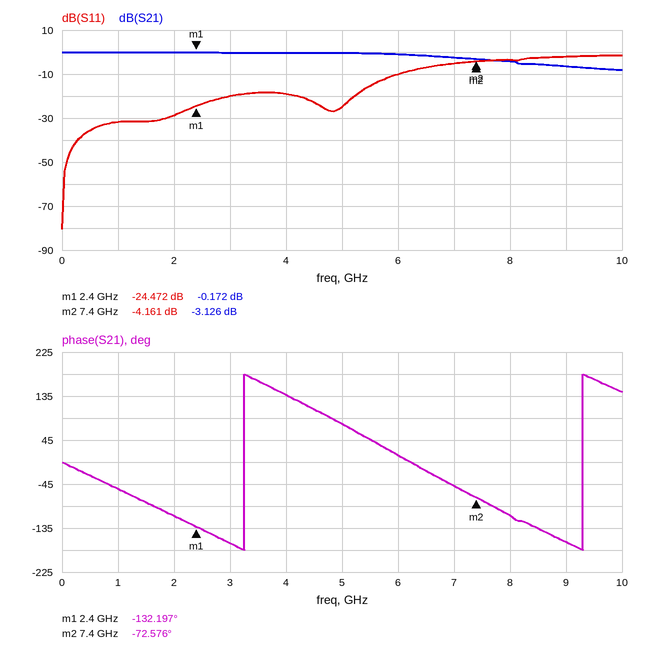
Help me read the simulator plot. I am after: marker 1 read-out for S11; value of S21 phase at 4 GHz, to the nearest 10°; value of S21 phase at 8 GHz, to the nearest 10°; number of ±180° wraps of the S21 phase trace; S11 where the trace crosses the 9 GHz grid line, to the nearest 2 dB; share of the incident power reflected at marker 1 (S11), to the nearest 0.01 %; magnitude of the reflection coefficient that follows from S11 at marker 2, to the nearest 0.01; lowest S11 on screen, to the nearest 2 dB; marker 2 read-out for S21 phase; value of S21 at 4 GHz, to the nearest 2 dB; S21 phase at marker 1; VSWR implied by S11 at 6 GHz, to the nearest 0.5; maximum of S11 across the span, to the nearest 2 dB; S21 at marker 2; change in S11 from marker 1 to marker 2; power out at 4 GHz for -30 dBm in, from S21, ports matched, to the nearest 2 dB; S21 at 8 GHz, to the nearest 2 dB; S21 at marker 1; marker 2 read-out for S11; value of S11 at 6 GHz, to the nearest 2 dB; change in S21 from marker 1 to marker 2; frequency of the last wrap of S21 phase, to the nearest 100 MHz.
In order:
-24.472 dB
140°
-110°
2
-2 dB
0.36 %
0.62
-80 dB
-72.576°
0 dB
-132.197°
2.0
-2 dB
-3.126 dB
20.311 dB
-30 dBm
-4 dB
-0.172 dB
-4.161 dB
-10 dB
-2.954 dB
9.3 GHz
